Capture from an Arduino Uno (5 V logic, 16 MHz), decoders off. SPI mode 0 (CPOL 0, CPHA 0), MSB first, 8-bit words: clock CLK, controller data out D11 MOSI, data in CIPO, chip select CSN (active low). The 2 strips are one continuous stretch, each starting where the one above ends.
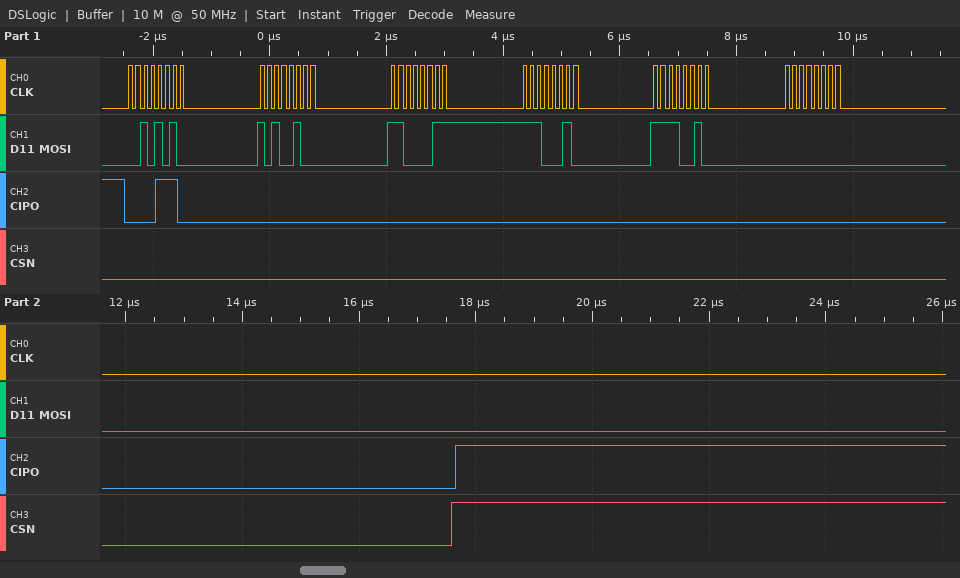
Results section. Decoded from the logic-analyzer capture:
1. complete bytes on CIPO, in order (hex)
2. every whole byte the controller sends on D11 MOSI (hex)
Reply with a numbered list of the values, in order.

1. 0E 00 00 00 00 00
2. 2A A4 C3 E2 F2 00
